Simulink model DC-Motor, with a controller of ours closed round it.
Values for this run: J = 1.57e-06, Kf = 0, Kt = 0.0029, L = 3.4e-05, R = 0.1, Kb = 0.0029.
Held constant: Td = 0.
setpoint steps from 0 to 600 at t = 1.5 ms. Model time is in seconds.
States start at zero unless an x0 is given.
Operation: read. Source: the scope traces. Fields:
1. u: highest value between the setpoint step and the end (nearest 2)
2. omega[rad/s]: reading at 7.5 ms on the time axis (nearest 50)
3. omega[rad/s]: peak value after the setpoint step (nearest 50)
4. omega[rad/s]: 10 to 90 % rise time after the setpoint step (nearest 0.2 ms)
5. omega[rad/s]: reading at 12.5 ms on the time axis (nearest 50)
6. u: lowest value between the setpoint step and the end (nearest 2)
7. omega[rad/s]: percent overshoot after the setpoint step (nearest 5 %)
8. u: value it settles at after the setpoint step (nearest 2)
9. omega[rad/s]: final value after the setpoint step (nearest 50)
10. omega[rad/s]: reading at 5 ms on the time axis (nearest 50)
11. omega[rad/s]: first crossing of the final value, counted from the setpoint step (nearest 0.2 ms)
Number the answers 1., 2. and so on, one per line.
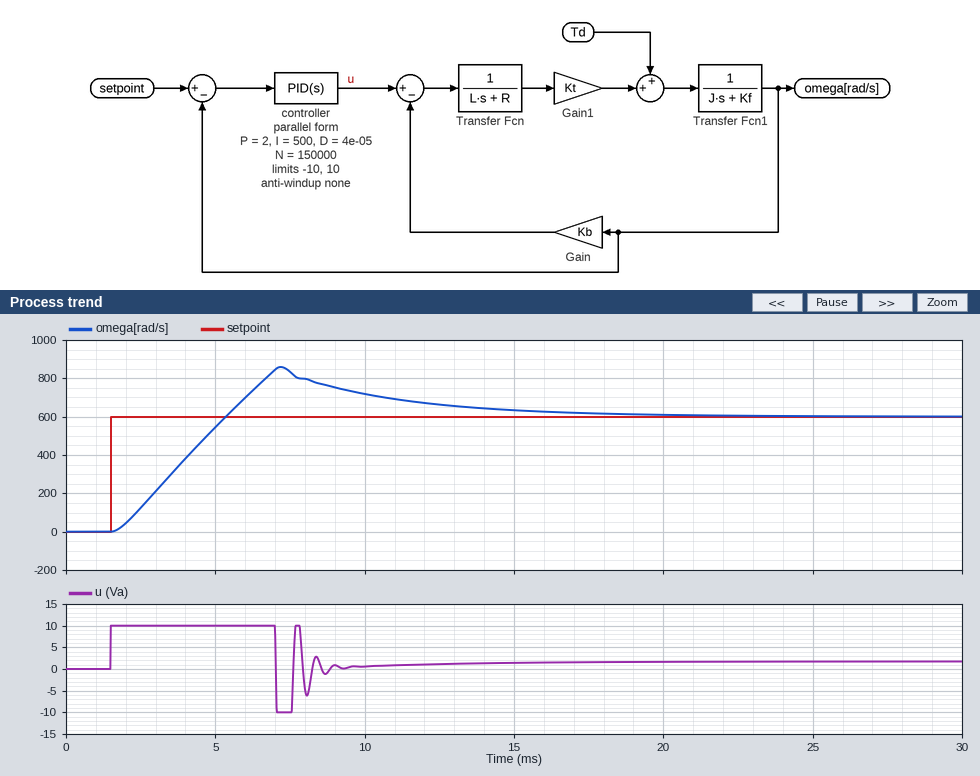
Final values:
1. 10
2. 850
3. 850
4. 2.8 ms
5. 650
6. -10
7. 45 %
8. 2
9. 600
10. 550
11. 3.8 ms
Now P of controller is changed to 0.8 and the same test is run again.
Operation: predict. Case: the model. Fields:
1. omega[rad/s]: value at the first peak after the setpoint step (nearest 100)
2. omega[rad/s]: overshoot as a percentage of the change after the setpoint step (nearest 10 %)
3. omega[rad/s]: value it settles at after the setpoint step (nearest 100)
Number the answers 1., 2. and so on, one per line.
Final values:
1. 1000
2. 70 %
3. 600
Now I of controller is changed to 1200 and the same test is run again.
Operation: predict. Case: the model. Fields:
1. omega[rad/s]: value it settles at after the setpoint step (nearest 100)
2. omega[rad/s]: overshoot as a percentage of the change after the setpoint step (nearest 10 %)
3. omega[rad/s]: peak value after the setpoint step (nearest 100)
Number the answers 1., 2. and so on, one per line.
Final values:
1. 600
2. 70 %
3. 1000
